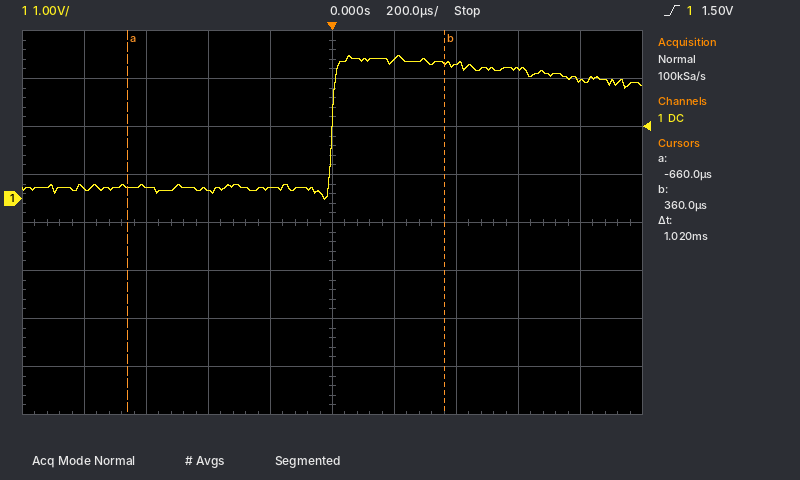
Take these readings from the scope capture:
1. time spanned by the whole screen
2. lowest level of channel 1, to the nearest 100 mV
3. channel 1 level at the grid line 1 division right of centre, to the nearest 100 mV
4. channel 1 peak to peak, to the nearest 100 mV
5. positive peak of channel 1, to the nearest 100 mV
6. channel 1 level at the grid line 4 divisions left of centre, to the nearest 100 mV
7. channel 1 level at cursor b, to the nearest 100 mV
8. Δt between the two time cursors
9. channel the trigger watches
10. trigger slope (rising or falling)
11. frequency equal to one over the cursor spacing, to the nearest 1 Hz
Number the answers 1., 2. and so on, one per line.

1. 2 ms
2. 0.0 V
3. 2.9 V
4. 3.0 V
5. 3.0 V
6. 200 mV
7. 2.8 V
8. 1.02 ms
9. channel 1
10. rising
11. 980 Hz
